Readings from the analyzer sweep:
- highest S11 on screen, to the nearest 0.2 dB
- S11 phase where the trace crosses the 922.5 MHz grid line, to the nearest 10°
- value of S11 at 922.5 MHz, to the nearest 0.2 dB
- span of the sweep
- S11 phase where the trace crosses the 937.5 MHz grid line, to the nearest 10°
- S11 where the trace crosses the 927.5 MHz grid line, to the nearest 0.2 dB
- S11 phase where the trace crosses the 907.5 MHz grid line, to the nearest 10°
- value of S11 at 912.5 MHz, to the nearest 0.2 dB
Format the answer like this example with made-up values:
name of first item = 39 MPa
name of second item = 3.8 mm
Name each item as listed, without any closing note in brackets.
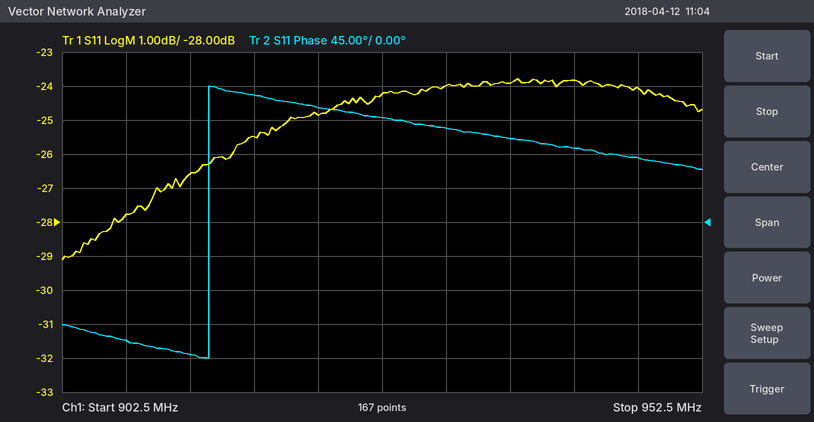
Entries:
highest S11 on screen, to the nearest 0.2 dB = -23.8 dB
S11 phase where the trace crosses the 922.5 MHz grid line, to the nearest 10° = 150°
value of S11 at 922.5 MHz, to the nearest 0.2 dB = -24.8 dB
span of the sweep = 50 MHz
S11 phase where the trace crosses the 937.5 MHz grid line, to the nearest 10° = 110°
S11 where the trace crosses the 927.5 MHz grid line, to the nearest 0.2 dB = -24.2 dB
S11 phase where the trace crosses the 907.5 MHz grid line, to the nearest 10° = -160°
value of S11 at 912.5 MHz, to the nearest 0.2 dB = -26.6 dB
